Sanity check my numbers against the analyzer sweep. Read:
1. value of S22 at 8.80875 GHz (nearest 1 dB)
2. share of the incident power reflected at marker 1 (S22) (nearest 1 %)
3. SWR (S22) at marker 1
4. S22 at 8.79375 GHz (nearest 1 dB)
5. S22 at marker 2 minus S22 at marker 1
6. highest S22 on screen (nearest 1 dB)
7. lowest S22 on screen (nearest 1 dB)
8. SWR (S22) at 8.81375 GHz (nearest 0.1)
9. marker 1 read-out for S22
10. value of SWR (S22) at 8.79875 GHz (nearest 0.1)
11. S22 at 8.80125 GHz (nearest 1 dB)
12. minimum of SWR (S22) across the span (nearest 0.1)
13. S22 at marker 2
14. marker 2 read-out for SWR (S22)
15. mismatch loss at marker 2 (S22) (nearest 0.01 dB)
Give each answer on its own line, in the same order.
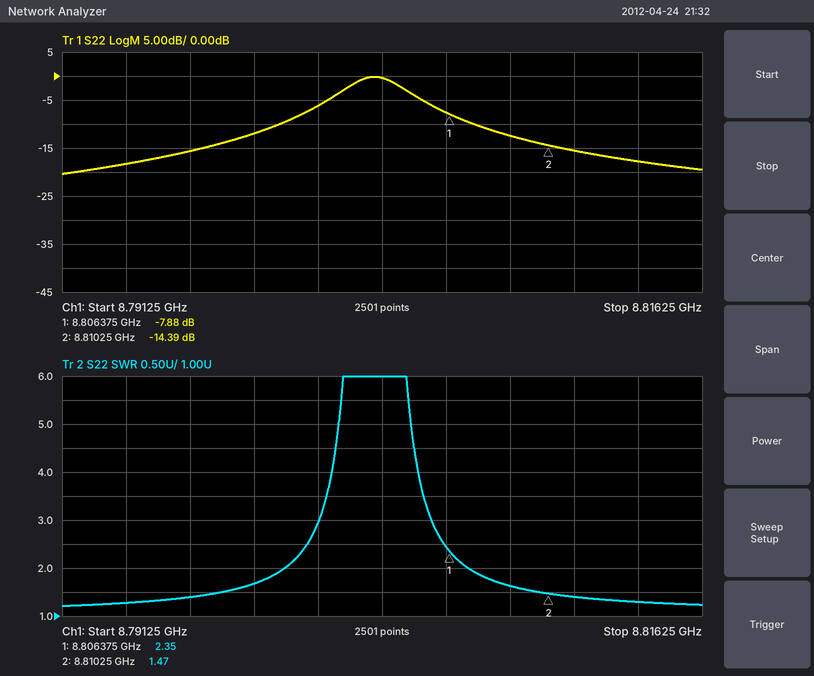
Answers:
-12 dB
16 %
2.35
-18 dB
-6.51 dB
0 dB
-20 dB
1.3
-7.88 dB
1.7
-6 dB
1.2
-14.39 dB
1.47
0.16 dB
